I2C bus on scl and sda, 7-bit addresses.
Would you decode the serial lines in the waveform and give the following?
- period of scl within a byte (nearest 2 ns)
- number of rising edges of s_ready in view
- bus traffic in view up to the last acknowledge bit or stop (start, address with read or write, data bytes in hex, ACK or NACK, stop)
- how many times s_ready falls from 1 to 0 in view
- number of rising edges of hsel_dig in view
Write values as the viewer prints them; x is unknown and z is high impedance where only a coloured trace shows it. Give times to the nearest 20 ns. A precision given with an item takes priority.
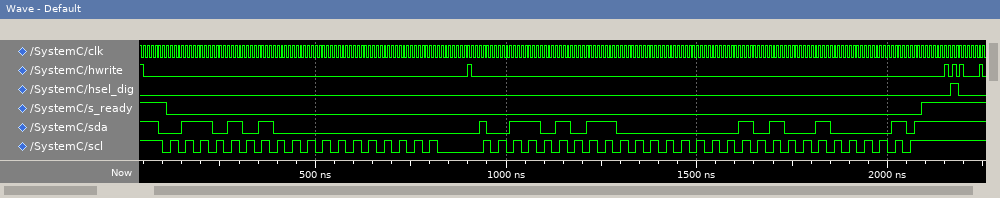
40 ns
1
start, address 35 write ACK, 00 ACK, repeated start, address 35 read ACK, 01 ACK, 90 NACK, stop
1
1
